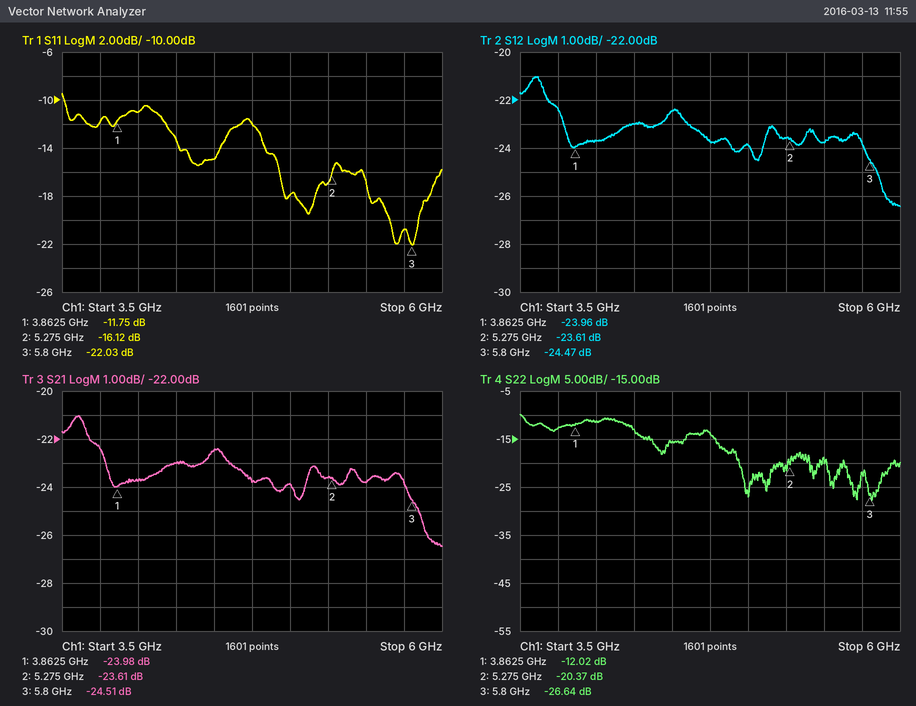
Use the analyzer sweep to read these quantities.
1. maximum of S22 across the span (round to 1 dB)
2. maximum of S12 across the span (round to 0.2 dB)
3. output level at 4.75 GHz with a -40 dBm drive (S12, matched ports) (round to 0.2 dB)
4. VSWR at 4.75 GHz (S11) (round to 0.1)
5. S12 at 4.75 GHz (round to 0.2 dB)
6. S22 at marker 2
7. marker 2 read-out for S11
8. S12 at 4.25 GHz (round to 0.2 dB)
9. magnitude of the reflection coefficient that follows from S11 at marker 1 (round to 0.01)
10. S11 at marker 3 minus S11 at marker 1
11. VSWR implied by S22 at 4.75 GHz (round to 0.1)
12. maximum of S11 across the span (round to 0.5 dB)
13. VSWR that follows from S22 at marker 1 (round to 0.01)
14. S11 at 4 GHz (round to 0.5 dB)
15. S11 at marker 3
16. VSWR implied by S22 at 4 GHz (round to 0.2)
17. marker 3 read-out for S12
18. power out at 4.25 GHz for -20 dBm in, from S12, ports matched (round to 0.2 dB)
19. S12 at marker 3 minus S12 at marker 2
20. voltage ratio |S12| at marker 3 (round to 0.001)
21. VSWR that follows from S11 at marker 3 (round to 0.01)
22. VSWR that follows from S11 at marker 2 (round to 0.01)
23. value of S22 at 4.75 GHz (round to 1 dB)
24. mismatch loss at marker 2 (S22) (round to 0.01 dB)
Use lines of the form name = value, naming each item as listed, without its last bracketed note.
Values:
maximum of S22 across the span = -10 dB
maximum of S12 across the span = -21.0 dB
output level at 4.75 GHz with a -40 dBm drive (S12, matched ports) = -63.8 dBm
VSWR at 4.75 GHz (S11) = 1.7
S12 at 4.75 GHz = -23.8 dB
S22 at marker 2 = -20.37 dB
marker 2 read-out for S11 = -16.12 dB
S12 at 4.25 GHz = -23.0 dB
magnitude of the reflection coefficient that follows from S11 at marker 1 = 0.26
S11 at marker 3 minus S11 at marker 1 = -10.28 dB
VSWR implied by S22 at 4.75 GHz = 1.5
maximum of S11 across the span = -9.5 dB
VSWR that follows from S22 at marker 1 = 1.67
S11 at 4 GHz = -11.0 dB
S11 at marker 3 = -22.03 dB
VSWR implied by S22 at 4 GHz = 1.8
marker 3 read-out for S12 = -24.47 dB
power out at 4.25 GHz for -20 dBm in, from S12, ports matched = -43.0 dBm
S12 at marker 3 minus S12 at marker 2 = -0.86 dB
voltage ratio |S12| at marker 3 = 0.060
VSWR that follows from S11 at marker 3 = 1.17
VSWR that follows from S11 at marker 2 = 1.37
value of S22 at 4.75 GHz = -14 dB
mismatch loss at marker 2 (S22) = 0.04 dB
